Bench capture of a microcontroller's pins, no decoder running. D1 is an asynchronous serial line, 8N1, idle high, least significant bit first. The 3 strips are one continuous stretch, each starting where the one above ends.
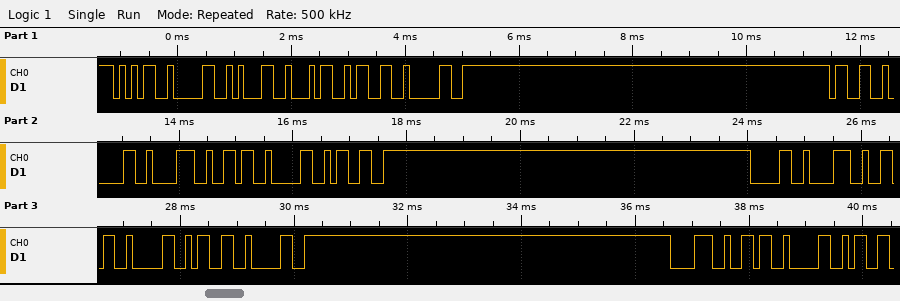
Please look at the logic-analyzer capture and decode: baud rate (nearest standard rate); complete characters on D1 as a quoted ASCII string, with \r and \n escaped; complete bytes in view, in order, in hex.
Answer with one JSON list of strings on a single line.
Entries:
["9600 baud", "\"501430308603086030860\"", "0x35 0x30 0x31 0x34 0x33 0x30 0x33 0x30 0x38 0x36 0x30 0x33 0x30 0x38 0x36 0x30 0x33 0x30 0x38 0x36 0x30"]
